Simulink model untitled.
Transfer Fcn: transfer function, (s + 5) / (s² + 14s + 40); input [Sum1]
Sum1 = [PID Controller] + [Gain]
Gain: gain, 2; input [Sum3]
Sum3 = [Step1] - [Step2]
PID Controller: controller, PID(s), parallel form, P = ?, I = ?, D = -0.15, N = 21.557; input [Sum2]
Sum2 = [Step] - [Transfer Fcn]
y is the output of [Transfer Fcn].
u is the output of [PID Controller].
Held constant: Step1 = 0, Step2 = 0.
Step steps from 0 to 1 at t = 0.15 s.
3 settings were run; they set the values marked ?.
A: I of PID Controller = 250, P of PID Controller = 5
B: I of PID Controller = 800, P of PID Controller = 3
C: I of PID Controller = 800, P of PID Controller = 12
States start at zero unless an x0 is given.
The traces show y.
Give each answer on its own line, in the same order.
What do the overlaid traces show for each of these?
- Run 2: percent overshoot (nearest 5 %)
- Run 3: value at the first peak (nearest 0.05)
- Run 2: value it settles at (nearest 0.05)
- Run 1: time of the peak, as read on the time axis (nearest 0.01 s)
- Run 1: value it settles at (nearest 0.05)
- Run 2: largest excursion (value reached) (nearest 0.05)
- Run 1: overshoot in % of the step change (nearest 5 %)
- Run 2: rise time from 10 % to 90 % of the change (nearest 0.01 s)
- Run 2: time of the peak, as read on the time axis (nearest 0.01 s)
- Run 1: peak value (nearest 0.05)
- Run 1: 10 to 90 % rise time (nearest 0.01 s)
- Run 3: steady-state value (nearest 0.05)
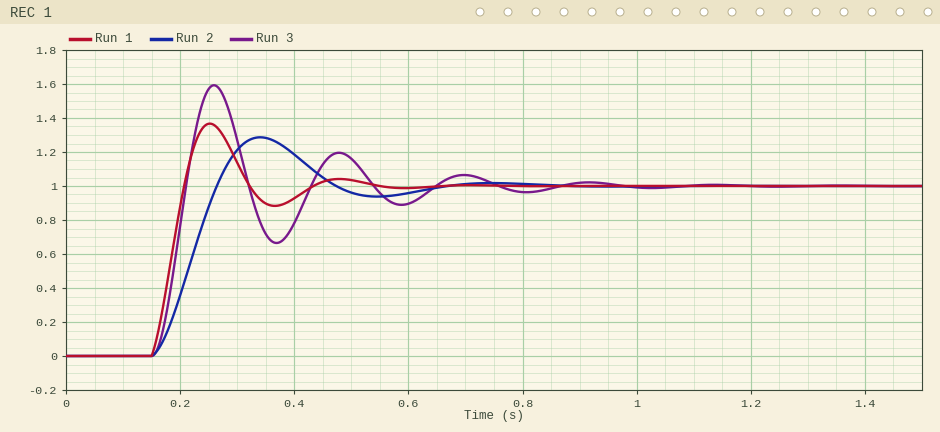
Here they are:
30 %
1.60
1.00
0.25 s
1.00
1.30
35 %
0.08 s
0.34 s
1.35
0.04 s
1.00
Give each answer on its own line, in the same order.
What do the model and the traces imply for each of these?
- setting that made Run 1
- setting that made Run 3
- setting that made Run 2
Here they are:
C
B
A
